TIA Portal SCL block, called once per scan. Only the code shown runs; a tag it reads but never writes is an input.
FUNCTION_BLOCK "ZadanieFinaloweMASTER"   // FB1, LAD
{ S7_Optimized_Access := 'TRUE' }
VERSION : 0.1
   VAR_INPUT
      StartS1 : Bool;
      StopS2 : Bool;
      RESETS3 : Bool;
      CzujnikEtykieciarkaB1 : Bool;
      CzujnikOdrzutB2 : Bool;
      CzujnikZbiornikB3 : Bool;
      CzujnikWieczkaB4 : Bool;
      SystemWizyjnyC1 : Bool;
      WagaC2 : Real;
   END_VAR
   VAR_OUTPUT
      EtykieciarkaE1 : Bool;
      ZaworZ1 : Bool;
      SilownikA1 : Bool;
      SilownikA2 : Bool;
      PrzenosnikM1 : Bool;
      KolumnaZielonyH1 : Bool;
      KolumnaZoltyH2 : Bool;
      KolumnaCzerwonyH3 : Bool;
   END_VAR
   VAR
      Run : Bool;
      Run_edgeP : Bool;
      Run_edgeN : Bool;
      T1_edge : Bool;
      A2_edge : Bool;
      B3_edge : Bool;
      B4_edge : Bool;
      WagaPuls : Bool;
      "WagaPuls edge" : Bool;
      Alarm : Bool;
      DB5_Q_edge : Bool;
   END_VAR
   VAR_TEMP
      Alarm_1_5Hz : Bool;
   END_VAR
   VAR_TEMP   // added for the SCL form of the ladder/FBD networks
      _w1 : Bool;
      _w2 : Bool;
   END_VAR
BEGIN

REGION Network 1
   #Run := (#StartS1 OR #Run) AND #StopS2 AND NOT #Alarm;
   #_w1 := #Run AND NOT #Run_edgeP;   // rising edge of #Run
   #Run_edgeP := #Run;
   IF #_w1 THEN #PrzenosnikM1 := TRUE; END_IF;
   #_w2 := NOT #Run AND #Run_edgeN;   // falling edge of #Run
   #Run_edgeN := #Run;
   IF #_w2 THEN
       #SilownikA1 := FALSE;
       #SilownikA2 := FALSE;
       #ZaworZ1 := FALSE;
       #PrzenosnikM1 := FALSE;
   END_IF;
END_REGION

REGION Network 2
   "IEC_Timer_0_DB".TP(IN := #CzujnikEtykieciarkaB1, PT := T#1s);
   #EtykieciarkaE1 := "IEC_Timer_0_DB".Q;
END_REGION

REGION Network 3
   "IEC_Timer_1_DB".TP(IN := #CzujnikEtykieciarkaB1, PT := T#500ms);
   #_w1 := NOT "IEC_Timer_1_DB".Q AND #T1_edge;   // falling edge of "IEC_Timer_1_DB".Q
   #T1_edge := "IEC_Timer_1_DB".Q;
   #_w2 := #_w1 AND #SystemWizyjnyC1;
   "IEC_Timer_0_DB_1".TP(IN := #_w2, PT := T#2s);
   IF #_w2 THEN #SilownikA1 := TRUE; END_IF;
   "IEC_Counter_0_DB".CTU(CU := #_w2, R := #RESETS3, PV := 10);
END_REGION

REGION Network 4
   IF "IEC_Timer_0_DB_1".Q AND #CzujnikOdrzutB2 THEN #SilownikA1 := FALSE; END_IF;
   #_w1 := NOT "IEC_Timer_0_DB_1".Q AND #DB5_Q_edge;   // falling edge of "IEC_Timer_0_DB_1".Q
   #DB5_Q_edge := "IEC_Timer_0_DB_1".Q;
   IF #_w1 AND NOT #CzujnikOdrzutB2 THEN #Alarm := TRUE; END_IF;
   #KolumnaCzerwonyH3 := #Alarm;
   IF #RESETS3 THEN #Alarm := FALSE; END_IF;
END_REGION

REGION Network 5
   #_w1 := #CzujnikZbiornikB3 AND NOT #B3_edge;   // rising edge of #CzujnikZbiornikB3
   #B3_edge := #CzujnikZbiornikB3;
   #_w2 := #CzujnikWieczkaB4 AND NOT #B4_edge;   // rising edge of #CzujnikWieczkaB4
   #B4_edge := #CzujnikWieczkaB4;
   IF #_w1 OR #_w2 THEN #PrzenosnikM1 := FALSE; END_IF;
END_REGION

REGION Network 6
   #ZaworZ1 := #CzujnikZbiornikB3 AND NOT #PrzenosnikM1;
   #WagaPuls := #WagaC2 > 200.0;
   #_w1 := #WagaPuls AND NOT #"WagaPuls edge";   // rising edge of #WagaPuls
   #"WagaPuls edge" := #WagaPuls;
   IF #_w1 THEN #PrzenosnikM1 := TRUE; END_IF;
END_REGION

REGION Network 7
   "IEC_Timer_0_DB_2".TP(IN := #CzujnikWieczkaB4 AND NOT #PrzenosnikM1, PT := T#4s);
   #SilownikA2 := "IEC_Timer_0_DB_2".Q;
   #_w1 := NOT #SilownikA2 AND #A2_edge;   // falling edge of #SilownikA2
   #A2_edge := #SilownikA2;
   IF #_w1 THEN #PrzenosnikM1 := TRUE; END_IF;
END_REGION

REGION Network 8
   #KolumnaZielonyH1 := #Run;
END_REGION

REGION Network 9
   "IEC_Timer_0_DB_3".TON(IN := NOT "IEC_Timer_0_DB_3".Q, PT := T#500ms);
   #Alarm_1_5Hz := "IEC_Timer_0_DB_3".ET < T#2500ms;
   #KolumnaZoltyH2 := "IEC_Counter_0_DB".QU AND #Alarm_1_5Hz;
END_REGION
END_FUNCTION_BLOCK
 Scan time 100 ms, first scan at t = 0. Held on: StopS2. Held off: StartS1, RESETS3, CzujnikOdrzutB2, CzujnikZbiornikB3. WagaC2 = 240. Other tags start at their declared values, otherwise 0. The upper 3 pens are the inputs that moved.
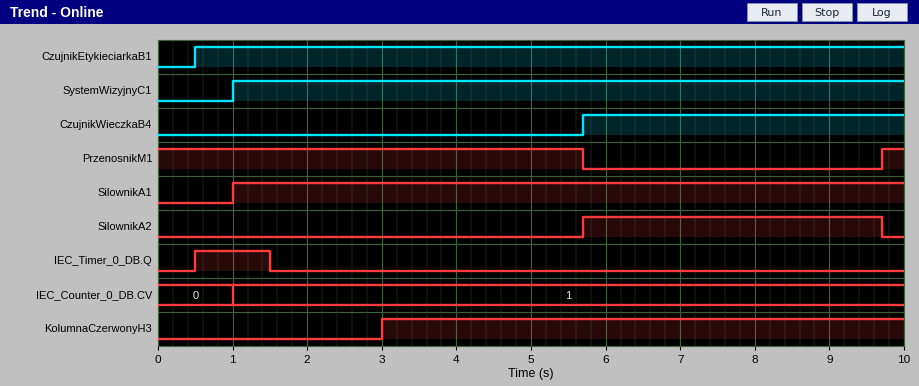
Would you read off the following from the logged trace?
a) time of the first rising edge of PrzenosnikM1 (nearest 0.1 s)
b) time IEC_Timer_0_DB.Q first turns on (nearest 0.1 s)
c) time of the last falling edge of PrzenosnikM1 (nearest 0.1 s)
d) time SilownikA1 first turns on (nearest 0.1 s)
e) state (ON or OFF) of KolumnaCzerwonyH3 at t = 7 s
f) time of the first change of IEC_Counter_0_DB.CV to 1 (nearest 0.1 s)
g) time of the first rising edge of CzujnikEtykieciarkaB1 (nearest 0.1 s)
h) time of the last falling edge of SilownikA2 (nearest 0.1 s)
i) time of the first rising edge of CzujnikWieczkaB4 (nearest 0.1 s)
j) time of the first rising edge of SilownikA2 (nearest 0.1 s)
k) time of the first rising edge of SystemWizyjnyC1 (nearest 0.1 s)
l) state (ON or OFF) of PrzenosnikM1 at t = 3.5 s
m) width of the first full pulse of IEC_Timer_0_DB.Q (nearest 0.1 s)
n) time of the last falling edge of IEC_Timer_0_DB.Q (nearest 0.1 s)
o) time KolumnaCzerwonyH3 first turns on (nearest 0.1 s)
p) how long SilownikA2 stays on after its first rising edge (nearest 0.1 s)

9.7 s
0.5 s
5.7 s
1.0 s
ON
1.0 s
0.5 s
9.7 s
5.7 s
5.7 s
1.0 s
ON
1.0 s
1.5 s
3.0 s
4.0 s
